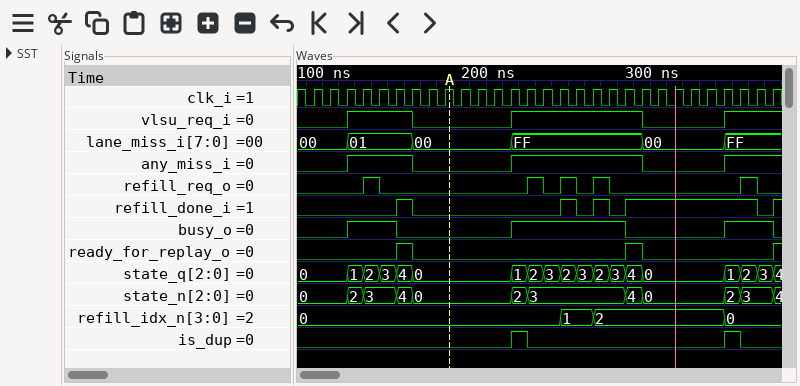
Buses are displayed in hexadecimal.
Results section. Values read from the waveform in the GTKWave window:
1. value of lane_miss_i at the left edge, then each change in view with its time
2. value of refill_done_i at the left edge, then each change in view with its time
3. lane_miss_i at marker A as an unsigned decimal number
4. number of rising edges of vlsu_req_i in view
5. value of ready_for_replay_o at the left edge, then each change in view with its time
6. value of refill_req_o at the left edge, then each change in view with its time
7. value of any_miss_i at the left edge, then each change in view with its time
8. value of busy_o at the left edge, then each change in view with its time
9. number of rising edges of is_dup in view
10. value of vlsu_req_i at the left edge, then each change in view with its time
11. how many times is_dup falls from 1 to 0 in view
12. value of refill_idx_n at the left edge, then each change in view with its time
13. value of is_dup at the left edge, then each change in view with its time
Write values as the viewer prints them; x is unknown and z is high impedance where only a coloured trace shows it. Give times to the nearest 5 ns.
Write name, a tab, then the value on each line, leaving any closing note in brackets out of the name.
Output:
value of lane_miss_i at the left edge, then each change in view with its time	00, 01 at 115 ns, 00 at 155 ns, FF at 215 ns, 00 at 295 ns, FF at 345 ns
value of refill_done_i at the left edge, then each change in view with its time	0, 1 at 145 ns, 0 at 155 ns, 1 at 245 ns, 0 at 255 ns, 1 at 265 ns, 0 at 275 ns, 1 at 285 ns, 0 at 365 ns, 1 at 375 ns
lane_miss_i at marker A as an unsigned decimal number	0
number of rising edges of vlsu_req_i in view	3
value of ready_for_replay_o at the left edge, then each change in view with its time	0, 1 at 145 ns, 0 at 155 ns, 1 at 285 ns, 0 at 295 ns, 1 at 375 ns
value of refill_req_o at the left edge, then each change in view with its time	0, 1 at 125 ns, 0 at 135 ns, 1 at 225 ns, 0 at 235 ns, 1 at 245 ns, 0 at 255 ns, 1 at 265 ns, 0 at 275 ns, 1 at 355 ns, 0 at 365 ns
value of any_miss_i at the left edge, then each change in view with its time	0, 1 at 115 ns, 0 at 155 ns, 1 at 215 ns, 0 at 295 ns, 1 at 345 ns
value of busy_o at the left edge, then each change in view with its time	0, 1 at 115 ns, 0 at 145 ns, 1 at 215 ns, 0 at 285 ns, 1 at 345 ns, 0 at 375 ns
number of rising edges of is_dup in view	2
value of vlsu_req_i at the left edge, then each change in view with its time	0, 1 at 115 ns, 0 at 155 ns, 1 at 215 ns, 0 at 295 ns, 1 at 345 ns
how many times is_dup falls from 1 to 0 in view	2
value of refill_idx_n at the left edge, then each change in view with its time	0, 1 at 245 ns, 2 at 265 ns, 0 at 345 ns
value of is_dup at the left edge, then each change in view with its time	0, 1 at 215 ns, 0 at 225 ns, 1 at 345 ns, 0 at 355 ns
